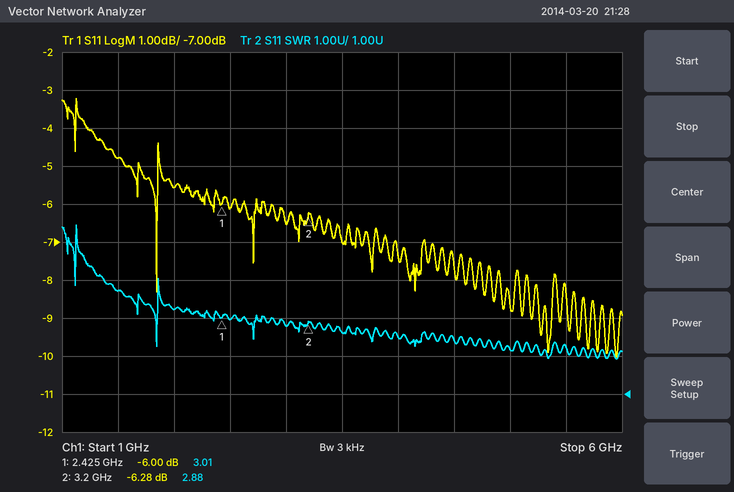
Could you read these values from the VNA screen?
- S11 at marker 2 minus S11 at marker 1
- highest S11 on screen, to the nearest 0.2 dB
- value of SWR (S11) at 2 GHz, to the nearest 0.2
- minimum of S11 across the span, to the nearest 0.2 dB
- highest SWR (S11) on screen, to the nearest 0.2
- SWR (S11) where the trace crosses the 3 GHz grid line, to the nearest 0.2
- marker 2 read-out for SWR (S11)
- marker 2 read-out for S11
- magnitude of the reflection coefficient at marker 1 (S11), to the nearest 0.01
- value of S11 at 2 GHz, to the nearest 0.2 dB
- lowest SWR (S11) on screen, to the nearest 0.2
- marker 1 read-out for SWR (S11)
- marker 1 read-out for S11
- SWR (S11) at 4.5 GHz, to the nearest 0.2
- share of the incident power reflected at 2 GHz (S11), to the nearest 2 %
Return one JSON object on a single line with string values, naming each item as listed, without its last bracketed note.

{"S11 at marker 2 minus S11 at marker 1": "-0.28 dB", "highest S11 on screen, to the nearest 0.2 dB": "-3.2 dB", "value of SWR (S11) at 2 GHz, to the nearest 0.2": "3.2", "minimum of S11 across the span, to the nearest 0.2 dB": "-10.0 dB", "highest SWR (S11) on screen, to the nearest 0.2": "5.4", "SWR (S11) where the trace crosses the 3 GHz grid line, to the nearest 0.2": "2.8", "marker 2 read-out for SWR": "2.88", "marker 2 read-out for S11": "-6.28 dB", "magnitude of the reflection coefficient at marker 1 (S11), to the nearest 0.01": "0.50", "value of S11 at 2 GHz, to the nearest 0.2 dB": "-5.6 dB", "lowest SWR (S11) on screen, to the nearest 0.2": "2.0", "marker 1 read-out for SWR": "3.01", "marker 1 read-out for S11": "-6.00 dB", "SWR (S11) at 4.5 GHz, to the nearest 0.2": "2.4", "share of the incident power reflected at 2 GHz (S11), to the nearest 2 %": "28 %"}
